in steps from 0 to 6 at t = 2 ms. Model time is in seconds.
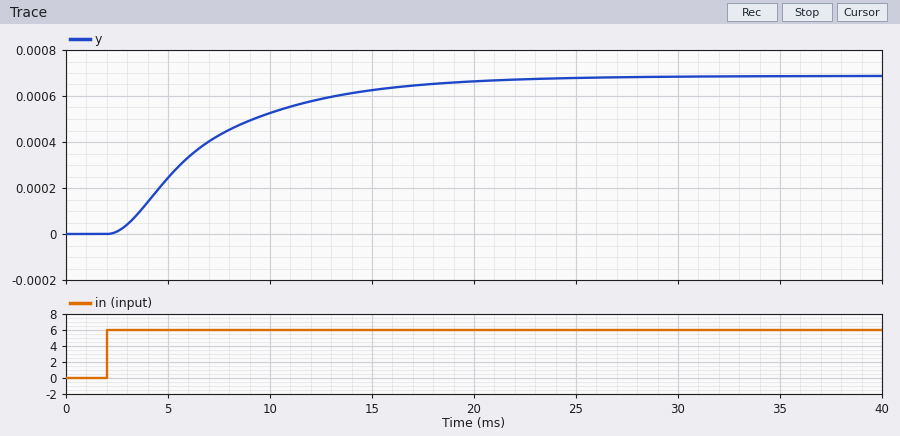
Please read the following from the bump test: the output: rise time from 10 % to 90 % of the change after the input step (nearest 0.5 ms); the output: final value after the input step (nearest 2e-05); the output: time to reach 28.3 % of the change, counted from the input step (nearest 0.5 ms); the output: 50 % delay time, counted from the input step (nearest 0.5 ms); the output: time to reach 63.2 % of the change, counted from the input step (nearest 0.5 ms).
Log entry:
11.0 ms
0.00068
2.5 ms
4.0 ms
5.5 ms
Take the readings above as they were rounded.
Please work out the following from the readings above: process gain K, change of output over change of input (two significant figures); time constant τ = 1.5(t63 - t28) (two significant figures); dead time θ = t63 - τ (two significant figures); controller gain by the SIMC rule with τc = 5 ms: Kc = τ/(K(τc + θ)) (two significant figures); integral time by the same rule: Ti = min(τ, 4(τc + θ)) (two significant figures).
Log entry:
0.00011
4.5 ms
1.0 ms
6800
4.5 ms
